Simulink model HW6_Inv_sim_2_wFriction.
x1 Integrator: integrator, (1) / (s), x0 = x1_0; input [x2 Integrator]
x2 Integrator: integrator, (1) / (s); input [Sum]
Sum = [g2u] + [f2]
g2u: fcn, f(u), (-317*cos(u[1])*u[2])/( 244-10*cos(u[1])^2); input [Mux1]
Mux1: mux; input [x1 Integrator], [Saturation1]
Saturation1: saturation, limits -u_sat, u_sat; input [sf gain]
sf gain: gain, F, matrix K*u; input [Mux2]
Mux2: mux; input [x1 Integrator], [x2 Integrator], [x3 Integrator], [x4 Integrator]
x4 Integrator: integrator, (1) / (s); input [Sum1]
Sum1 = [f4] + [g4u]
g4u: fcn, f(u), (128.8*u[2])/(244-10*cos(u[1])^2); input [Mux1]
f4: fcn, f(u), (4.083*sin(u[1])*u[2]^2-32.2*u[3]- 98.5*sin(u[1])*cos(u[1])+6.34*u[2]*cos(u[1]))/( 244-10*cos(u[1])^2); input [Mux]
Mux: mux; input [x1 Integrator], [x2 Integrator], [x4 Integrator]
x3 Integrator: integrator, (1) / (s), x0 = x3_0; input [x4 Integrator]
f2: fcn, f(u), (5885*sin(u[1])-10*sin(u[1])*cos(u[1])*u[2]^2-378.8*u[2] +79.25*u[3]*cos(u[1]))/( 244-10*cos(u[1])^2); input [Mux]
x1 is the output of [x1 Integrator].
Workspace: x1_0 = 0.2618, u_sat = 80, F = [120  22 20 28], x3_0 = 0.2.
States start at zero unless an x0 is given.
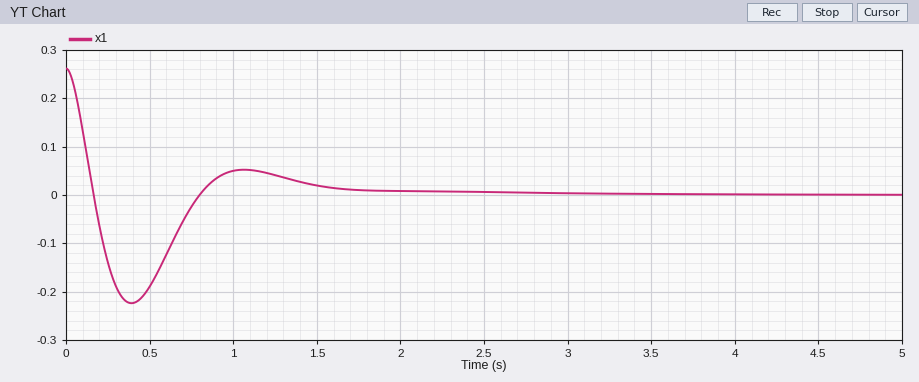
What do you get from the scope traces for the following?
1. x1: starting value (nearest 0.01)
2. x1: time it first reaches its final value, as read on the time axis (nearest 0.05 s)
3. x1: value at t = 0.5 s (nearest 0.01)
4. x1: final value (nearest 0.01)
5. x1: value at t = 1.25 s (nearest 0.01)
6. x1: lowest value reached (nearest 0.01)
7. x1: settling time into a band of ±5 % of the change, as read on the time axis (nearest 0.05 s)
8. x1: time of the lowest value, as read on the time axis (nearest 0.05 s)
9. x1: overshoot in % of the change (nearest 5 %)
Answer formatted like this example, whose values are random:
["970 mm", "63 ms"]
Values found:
["0.26", "0.15 s", "-0.19", "0.00", "0.04", "-0.22", "1.65 s", "0.40 s", "85 %"]
